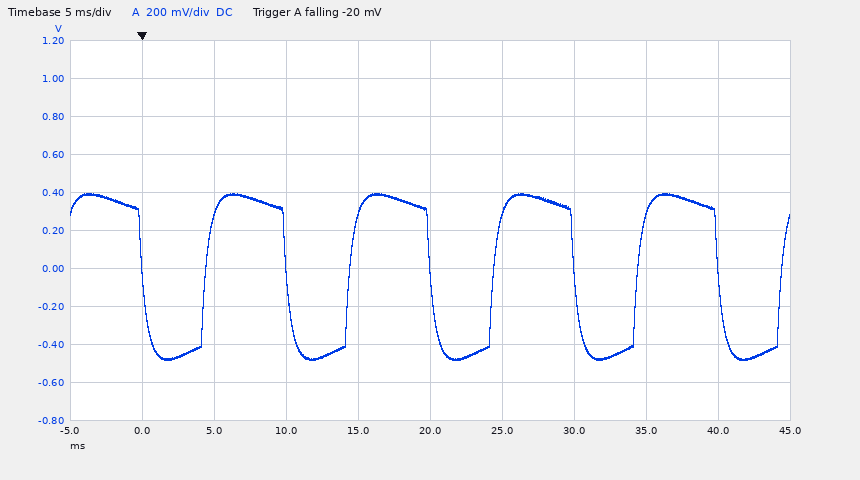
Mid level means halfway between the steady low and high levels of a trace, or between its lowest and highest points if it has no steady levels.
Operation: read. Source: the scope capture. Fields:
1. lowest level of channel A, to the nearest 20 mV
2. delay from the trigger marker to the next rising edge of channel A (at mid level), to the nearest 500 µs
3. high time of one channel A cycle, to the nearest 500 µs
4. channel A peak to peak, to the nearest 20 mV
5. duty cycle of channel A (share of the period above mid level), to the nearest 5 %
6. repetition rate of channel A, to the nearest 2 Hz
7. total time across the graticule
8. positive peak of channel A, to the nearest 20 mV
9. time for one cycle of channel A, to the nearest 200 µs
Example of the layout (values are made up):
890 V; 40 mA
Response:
-480 mV; 4.5 ms; 5.5 ms; 880 mV; 55 %; 100 Hz; 50 ms; 400 mV; 10.0 ms
